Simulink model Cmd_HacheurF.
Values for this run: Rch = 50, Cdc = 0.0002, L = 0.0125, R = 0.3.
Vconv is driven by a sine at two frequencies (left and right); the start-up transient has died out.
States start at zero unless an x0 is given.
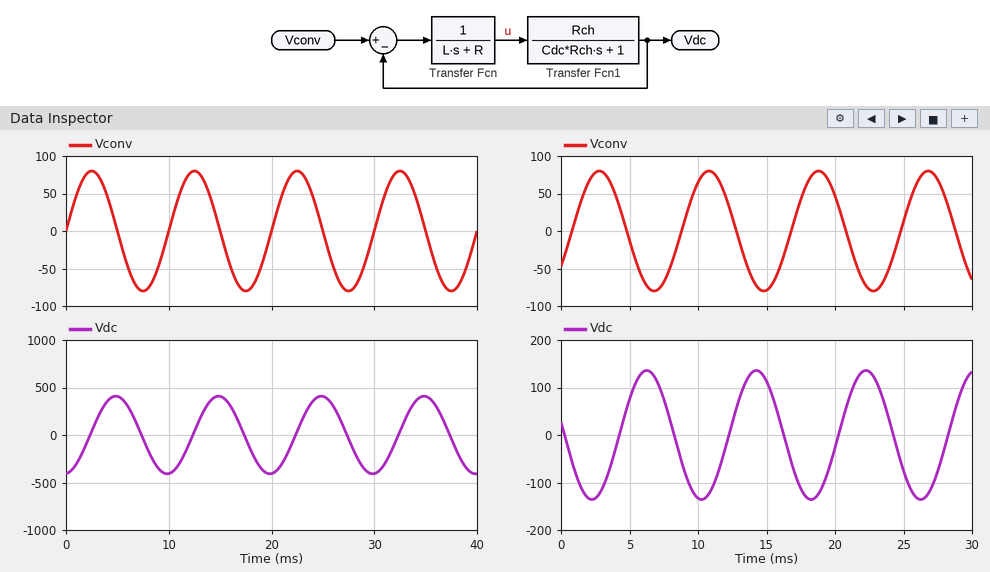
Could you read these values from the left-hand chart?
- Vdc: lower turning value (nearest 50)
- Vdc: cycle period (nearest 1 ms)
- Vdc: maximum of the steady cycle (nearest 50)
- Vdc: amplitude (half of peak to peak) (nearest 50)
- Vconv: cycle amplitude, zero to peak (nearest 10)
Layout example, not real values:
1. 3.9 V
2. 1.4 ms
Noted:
1. -400
2. 10 ms
3. 400
4. 400
5. 80
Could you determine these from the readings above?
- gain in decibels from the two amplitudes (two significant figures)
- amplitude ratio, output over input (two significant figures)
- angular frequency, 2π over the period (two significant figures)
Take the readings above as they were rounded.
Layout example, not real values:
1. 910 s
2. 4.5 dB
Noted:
1. 14 dB
2. 5.0
3. 0.63 rad/ms
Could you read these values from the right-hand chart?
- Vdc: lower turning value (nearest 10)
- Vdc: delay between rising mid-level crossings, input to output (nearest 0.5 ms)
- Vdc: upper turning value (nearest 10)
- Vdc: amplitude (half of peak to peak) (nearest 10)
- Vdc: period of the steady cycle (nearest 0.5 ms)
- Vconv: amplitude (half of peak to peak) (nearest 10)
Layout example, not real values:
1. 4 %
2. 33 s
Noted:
1. -140
2. 3.5 ms
3. 140
4. 140
5. 8.0 ms
6. 80
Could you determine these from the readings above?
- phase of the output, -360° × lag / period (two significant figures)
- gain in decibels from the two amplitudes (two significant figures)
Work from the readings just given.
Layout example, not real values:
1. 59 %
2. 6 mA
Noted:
1. -160°
2. 4.9 dB
